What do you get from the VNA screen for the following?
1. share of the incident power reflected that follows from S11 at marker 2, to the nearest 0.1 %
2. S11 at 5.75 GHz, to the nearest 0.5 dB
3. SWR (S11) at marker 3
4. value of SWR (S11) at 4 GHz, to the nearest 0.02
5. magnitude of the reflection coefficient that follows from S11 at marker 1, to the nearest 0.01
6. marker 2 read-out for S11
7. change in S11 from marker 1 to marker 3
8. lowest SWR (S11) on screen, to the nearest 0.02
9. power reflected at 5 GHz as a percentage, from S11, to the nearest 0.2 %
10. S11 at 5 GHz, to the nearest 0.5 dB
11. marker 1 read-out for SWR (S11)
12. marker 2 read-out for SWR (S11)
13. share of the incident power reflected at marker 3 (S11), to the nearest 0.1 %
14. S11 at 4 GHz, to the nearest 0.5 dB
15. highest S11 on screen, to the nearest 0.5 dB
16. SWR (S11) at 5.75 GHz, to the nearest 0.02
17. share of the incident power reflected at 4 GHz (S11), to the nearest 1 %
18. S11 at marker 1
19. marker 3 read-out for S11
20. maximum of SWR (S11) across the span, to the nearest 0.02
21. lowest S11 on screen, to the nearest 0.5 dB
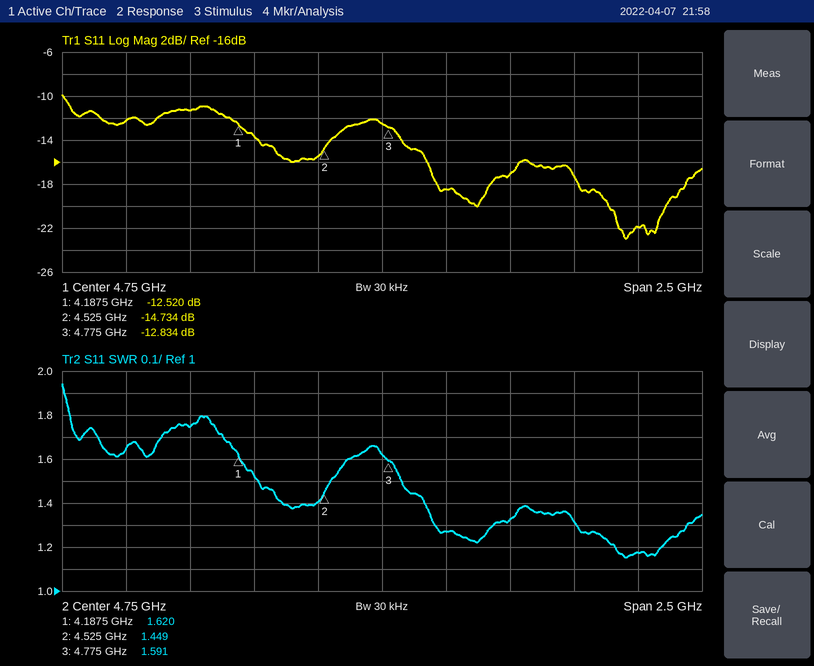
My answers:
3.4 %
-22.0 dB
1.591
1.74
0.24
-14.734 dB
-0.314 dB
1.16
1.4 %
-18.5 dB
1.620
1.449
5.2 %
-11.5 dB
-10.0 dB
1.18
7 %
-12.520 dB
-12.834 dB
1.94
-23.0 dB
